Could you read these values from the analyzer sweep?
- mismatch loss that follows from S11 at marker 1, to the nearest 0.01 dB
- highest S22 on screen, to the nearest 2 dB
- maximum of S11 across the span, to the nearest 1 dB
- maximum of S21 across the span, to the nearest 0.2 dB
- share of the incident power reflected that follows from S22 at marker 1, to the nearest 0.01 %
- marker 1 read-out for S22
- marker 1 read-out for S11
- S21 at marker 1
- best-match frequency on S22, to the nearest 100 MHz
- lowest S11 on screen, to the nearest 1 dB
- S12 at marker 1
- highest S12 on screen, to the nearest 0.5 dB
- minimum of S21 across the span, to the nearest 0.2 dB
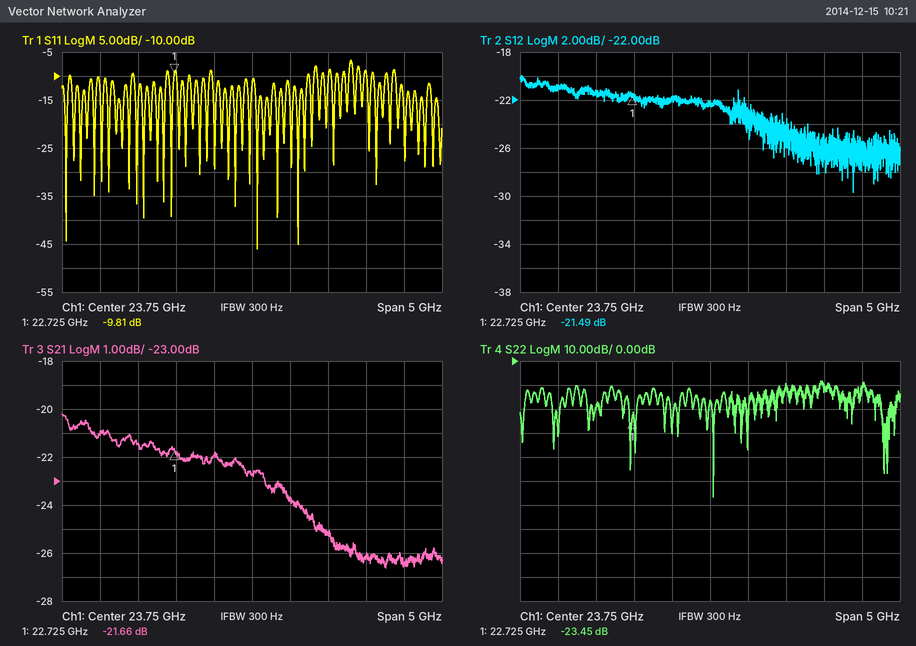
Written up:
0.48 dB
-8 dB
-7 dB
-20.2 dB
0.45 %
-23.45 dB
-9.81 dB
-21.66 dB
23.8 GHz
-46 dB
-21.49 dB
-20.0 dB
-26.6 dB
